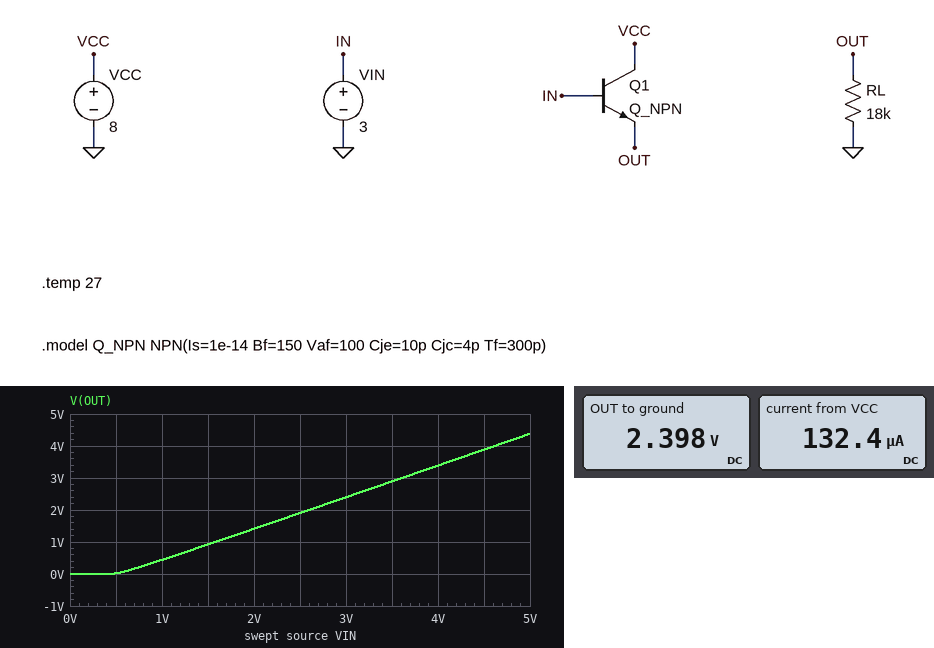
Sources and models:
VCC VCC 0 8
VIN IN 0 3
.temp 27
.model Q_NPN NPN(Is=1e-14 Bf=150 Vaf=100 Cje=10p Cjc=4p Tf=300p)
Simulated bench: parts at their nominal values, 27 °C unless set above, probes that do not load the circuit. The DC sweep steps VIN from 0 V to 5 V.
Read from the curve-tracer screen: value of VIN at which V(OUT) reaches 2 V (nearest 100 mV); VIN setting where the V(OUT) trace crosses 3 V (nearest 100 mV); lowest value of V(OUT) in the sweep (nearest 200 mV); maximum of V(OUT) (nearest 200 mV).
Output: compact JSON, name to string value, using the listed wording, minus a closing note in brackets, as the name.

{"value of VIN at which V(OUT) reaches 2 V": "2.6 V", "VIN setting where the V(OUT) trace crosses 3 V": "3.6 V", "lowest value of V(OUT) in the sweep": "0 V", "maximum of V(OUT)": "4.4 V"}
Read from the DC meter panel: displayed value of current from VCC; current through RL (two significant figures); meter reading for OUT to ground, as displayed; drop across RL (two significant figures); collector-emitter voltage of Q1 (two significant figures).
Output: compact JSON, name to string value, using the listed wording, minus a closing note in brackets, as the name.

{"displayed value of current from VCC": "132.4 µA", "current through RL": "130 µA", "meter reading for OUT to ground, as displayed": "2.398 V", "drop across RL": "2.4 V", "collector-emitter voltage of Q1": "5.6 V"}
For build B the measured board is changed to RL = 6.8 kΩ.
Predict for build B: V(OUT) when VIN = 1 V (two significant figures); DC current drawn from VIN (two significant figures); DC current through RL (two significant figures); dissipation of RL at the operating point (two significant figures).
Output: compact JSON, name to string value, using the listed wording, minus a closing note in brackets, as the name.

{"V(OUT) when VIN = 1 V": "420 mV", "DC current drawn from VIN": "2.2 µA", "DC current through RL": "350 µA", "dissipation of RL at the operating point": "830 µW"}
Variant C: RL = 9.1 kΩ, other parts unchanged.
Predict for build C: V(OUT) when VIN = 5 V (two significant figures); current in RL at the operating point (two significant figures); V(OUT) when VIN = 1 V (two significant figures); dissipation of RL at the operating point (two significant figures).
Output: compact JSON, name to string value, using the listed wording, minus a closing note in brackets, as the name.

{"V(OUT) when VIN = 5 V": "4.4 V", "current in RL at the operating point": "260 µA", "V(OUT) when VIN = 1 V": "430 mV", "dissipation of RL at the operating point": "620 µW"}
